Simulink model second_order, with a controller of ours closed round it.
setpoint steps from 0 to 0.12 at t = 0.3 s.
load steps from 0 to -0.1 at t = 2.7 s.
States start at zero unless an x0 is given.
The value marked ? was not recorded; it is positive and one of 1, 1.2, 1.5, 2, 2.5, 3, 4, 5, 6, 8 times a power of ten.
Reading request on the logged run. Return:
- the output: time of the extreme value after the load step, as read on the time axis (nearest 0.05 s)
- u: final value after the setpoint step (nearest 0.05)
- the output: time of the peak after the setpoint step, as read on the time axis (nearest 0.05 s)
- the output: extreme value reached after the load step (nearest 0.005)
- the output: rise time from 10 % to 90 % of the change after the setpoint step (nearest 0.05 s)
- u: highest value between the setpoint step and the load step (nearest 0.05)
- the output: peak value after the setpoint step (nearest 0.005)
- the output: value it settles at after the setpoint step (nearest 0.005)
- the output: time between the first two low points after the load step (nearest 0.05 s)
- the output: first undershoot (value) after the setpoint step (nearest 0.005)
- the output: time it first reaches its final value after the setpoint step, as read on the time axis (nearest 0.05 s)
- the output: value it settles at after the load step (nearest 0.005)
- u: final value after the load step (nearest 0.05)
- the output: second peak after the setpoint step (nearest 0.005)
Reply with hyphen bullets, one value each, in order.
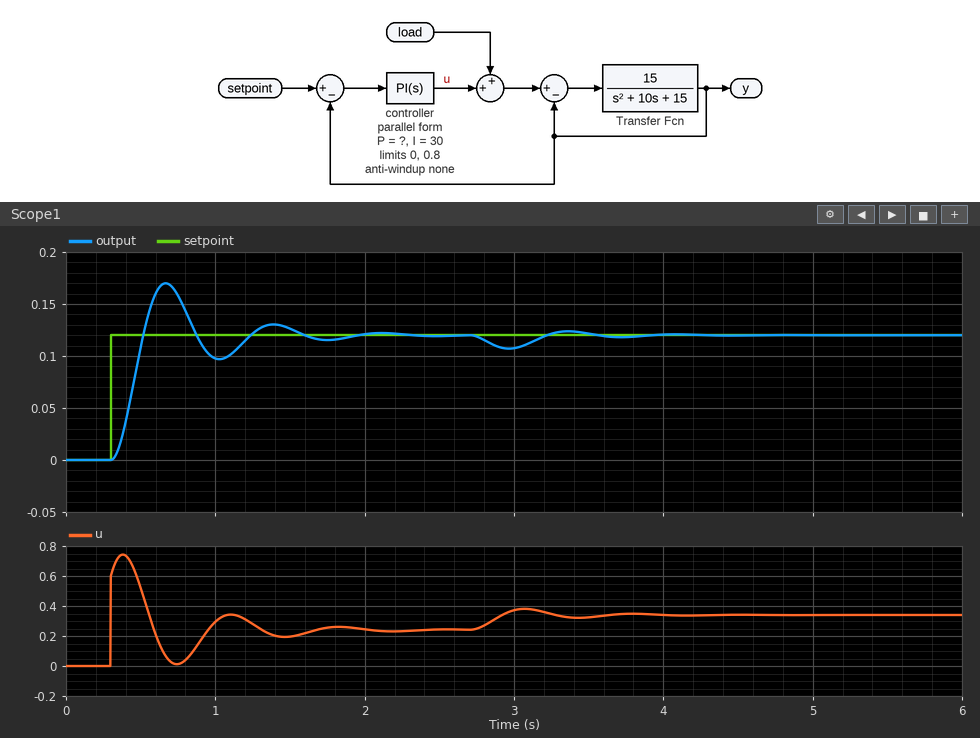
- 2.95 s
- 0.25
- 0.65 s
- 0.105
- 0.15 s
- 0.75
- 0.170
- 0.120
- 0.75 s
- 0.095
- 0.50 s
- 0.120
- 0.35
- 0.130
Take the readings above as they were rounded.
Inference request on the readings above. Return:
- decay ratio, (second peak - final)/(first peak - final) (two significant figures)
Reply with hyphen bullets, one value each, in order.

- 0.20
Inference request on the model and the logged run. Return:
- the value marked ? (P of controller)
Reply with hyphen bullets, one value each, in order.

- 5
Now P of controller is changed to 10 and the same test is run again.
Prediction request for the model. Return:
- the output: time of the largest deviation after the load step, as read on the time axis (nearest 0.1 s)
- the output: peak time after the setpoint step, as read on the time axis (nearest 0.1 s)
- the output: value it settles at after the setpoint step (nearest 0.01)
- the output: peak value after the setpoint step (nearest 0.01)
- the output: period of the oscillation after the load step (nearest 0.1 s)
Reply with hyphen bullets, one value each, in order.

- 2.9 s
- 0.6 s
- 0.12
- 0.16
- 0.5 s
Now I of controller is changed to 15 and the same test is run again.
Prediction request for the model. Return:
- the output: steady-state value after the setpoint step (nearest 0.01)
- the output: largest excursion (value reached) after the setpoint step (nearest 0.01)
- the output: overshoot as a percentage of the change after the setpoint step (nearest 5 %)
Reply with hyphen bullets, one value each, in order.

- 0.12
- 0.14
- 15 %
